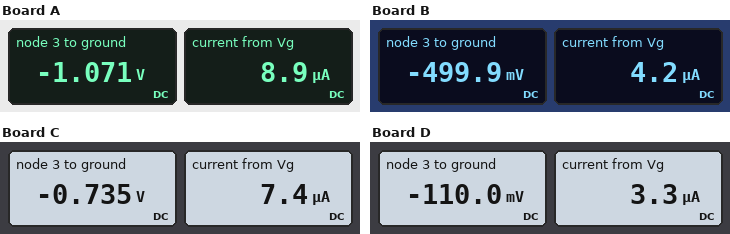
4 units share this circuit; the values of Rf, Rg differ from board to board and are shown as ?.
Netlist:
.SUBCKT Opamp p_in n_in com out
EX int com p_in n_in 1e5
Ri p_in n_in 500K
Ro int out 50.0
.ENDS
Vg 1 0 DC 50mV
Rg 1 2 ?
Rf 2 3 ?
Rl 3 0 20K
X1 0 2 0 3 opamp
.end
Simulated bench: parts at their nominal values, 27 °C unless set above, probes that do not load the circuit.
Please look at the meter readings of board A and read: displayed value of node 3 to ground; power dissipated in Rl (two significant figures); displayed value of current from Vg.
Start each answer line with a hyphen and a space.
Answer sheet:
- -1.071 V
- 57 µW
- 8.9 µA
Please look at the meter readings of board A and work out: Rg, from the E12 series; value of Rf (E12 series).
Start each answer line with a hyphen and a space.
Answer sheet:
- 5.6 kΩ
- 120 kΩ
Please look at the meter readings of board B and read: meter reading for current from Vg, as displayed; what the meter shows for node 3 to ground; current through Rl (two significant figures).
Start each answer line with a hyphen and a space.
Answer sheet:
- 4.2 µA
- -499.9 mV
- 25 µA
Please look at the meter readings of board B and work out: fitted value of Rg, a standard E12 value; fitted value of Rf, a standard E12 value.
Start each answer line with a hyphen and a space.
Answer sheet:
- 12 kΩ
- 120 kΩ
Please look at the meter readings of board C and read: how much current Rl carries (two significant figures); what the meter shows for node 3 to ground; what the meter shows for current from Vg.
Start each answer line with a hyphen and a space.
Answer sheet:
- 37 µA
- -0.735 V
- 7.4 µA
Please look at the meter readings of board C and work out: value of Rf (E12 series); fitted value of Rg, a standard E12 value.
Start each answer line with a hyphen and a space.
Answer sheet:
- 100 kΩ
- 6.8 kΩ
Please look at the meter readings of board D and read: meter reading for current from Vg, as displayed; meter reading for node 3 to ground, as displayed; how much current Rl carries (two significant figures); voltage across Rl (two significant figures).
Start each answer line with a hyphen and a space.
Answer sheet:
- 3.3 µA
- -110.0 mV
- 5.5 µA
- 110 mV
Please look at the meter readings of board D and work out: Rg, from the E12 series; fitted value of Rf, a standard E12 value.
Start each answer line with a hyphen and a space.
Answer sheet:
- 15 kΩ
- 33 kΩ
